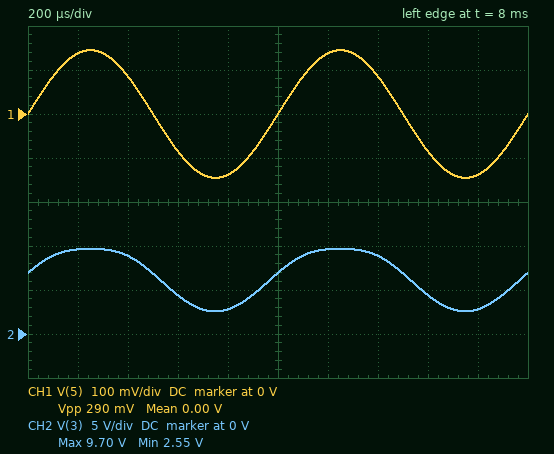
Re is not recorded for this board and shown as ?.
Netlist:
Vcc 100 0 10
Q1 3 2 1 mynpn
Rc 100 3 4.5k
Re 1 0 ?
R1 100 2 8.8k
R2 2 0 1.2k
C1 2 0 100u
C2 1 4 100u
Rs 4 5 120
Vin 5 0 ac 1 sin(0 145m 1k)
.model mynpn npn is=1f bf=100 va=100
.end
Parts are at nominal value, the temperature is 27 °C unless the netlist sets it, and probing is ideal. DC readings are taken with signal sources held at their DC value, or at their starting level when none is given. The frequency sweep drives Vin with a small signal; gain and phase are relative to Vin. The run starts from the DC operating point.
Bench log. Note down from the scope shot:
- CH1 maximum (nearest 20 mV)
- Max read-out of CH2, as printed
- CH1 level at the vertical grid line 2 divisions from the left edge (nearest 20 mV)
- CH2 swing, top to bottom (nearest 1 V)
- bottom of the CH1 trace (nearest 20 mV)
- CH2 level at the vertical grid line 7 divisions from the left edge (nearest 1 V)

140 mV
9.70 V
80 mV
7 V
-140 mV
9 V
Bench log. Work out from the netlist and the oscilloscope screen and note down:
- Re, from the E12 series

680 Ω
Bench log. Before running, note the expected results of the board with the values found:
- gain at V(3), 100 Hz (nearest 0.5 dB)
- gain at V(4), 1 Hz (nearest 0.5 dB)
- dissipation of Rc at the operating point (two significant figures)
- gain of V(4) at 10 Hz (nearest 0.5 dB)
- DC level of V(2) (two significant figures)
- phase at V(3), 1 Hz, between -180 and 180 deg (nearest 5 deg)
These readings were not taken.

28.5 dB
0 dB
2.3 mW
-2.5 dB
1.2 V
85 deg
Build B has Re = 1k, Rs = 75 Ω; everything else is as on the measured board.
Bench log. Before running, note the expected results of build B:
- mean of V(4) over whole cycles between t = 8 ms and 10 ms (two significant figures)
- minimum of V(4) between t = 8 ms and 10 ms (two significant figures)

9.9 mV
-49 mV
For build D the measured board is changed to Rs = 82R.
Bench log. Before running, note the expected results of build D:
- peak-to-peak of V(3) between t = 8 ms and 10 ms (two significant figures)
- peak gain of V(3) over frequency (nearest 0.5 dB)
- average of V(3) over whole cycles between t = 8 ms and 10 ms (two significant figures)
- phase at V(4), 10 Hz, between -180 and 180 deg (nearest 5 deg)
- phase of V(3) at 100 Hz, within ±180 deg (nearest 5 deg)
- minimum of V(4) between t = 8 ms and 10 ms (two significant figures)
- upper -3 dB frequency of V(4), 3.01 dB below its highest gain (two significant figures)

8.8 V
31.0 dB
6.3 V
-25 deg
10 deg
-38 mV
15 Hz
